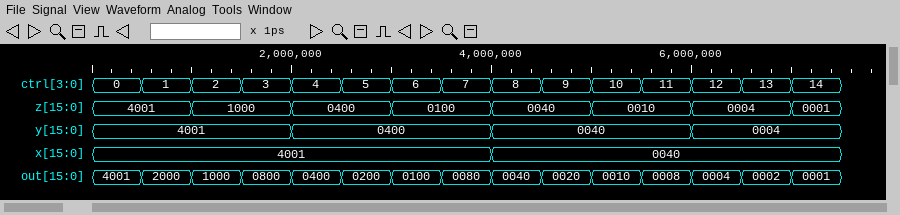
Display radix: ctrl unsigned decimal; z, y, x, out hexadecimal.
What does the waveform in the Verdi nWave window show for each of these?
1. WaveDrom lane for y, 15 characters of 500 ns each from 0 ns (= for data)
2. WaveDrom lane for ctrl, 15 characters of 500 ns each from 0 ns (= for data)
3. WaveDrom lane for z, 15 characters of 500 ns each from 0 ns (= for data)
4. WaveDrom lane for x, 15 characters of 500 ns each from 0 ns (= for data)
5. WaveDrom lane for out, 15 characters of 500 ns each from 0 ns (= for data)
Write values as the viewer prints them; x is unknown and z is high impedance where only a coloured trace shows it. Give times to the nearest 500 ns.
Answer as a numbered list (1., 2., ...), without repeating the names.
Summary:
1. {name: 'y', wave: '=...=...=...=..', data: '4001 0400 0040 0004'}
2. {name: 'ctrl', wave: '===============', data: '0 1 2 3 4 5 6 7 8 9 10 11 12 13 14'}
3. {name: 'z', wave: '=.=.=.=.=.=.=.=', data: '4001 1000 0400 0100 0040 0010 0004 0001'}
4. {name: 'x', wave: '=.......=......', data: '4001 0040'}
5. {name: 'out', wave: '===============', data: '4001 2000 1000 0800 0400 0200 0100 0080 0040 0020 0010 0008 0004 0002 0001'}
